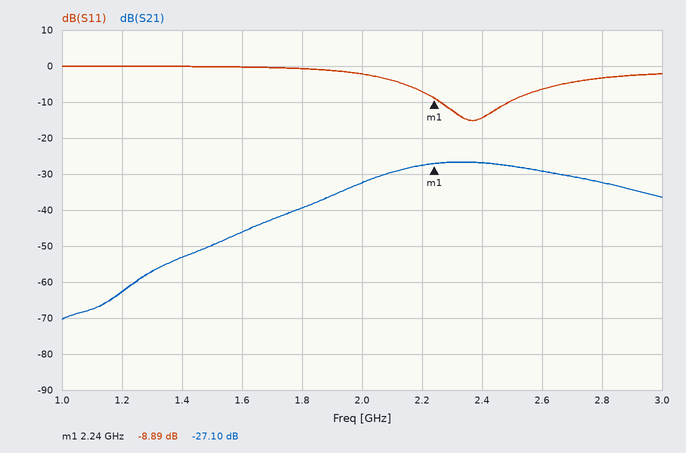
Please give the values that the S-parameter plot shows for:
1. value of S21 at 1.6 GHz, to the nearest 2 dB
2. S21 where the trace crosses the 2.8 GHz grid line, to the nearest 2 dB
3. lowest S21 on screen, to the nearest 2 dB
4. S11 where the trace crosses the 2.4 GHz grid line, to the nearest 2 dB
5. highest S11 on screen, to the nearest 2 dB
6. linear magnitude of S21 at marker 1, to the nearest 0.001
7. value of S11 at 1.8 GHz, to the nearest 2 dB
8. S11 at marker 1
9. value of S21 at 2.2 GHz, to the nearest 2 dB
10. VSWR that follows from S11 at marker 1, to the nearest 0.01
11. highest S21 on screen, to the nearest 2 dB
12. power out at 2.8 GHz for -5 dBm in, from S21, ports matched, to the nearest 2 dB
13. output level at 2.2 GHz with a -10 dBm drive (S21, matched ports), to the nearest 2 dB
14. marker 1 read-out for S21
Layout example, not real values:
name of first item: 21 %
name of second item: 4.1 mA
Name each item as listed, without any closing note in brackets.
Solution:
value of S21 at 1.6 GHz, to the nearest 2 dB: -46 dB
S21 where the trace crosses the 2.8 GHz grid line, to the nearest 2 dB: -32 dB
lowest S21 on screen, to the nearest 2 dB: -70 dB
S11 where the trace crosses the 2.4 GHz grid line, to the nearest 2 dB: -14 dB
highest S11 on screen, to the nearest 2 dB: 0 dB
linear magnitude of S21 at marker 1, to the nearest 0.001: 0.044
value of S11 at 1.8 GHz, to the nearest 2 dB: 0 dB
S11 at marker 1: -8.89 dB
value of S21 at 2.2 GHz, to the nearest 2 dB: -28 dB
VSWR that follows from S11 at marker 1, to the nearest 0.01: 2.12
highest S21 on screen, to the nearest 2 dB: -26 dB
power out at 2.8 GHz for -5 dBm in, from S21, ports matched, to the nearest 2 dB: -38 dBm
output level at 2.2 GHz with a -10 dBm drive (S21, matched ports), to the nearest 2 dB: -38 dBm
marker 1 read-out for S21: -27.10 dB
